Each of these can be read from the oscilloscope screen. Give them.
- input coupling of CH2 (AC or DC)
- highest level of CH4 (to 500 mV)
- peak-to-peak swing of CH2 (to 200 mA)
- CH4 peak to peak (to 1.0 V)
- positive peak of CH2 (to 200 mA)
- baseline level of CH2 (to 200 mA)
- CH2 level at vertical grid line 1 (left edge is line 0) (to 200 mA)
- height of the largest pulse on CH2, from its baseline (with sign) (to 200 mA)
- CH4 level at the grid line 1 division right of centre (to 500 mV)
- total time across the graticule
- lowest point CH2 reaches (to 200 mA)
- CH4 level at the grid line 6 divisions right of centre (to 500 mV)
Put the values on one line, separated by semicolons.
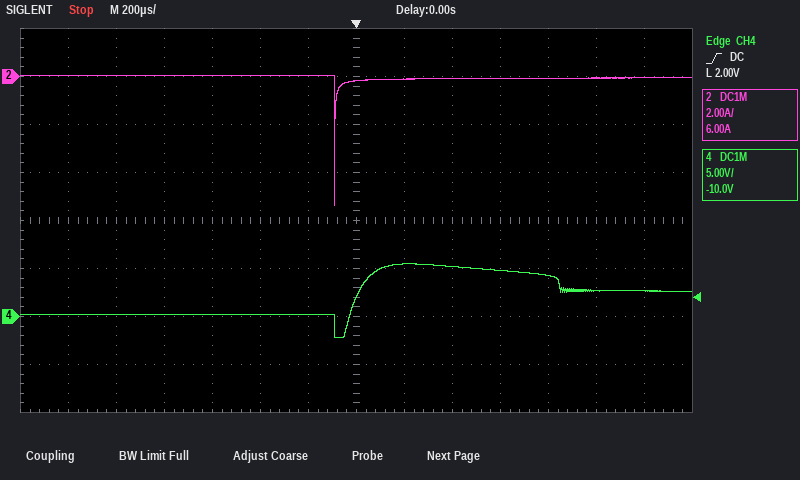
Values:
DC; 5.5 V; 5.4 A; 8.0 V; 0.0 A; 0.0 A; 0.0 A; -5.4 A; 5.5 V; 2.8 ms; -5.4 A; 2.5 V
